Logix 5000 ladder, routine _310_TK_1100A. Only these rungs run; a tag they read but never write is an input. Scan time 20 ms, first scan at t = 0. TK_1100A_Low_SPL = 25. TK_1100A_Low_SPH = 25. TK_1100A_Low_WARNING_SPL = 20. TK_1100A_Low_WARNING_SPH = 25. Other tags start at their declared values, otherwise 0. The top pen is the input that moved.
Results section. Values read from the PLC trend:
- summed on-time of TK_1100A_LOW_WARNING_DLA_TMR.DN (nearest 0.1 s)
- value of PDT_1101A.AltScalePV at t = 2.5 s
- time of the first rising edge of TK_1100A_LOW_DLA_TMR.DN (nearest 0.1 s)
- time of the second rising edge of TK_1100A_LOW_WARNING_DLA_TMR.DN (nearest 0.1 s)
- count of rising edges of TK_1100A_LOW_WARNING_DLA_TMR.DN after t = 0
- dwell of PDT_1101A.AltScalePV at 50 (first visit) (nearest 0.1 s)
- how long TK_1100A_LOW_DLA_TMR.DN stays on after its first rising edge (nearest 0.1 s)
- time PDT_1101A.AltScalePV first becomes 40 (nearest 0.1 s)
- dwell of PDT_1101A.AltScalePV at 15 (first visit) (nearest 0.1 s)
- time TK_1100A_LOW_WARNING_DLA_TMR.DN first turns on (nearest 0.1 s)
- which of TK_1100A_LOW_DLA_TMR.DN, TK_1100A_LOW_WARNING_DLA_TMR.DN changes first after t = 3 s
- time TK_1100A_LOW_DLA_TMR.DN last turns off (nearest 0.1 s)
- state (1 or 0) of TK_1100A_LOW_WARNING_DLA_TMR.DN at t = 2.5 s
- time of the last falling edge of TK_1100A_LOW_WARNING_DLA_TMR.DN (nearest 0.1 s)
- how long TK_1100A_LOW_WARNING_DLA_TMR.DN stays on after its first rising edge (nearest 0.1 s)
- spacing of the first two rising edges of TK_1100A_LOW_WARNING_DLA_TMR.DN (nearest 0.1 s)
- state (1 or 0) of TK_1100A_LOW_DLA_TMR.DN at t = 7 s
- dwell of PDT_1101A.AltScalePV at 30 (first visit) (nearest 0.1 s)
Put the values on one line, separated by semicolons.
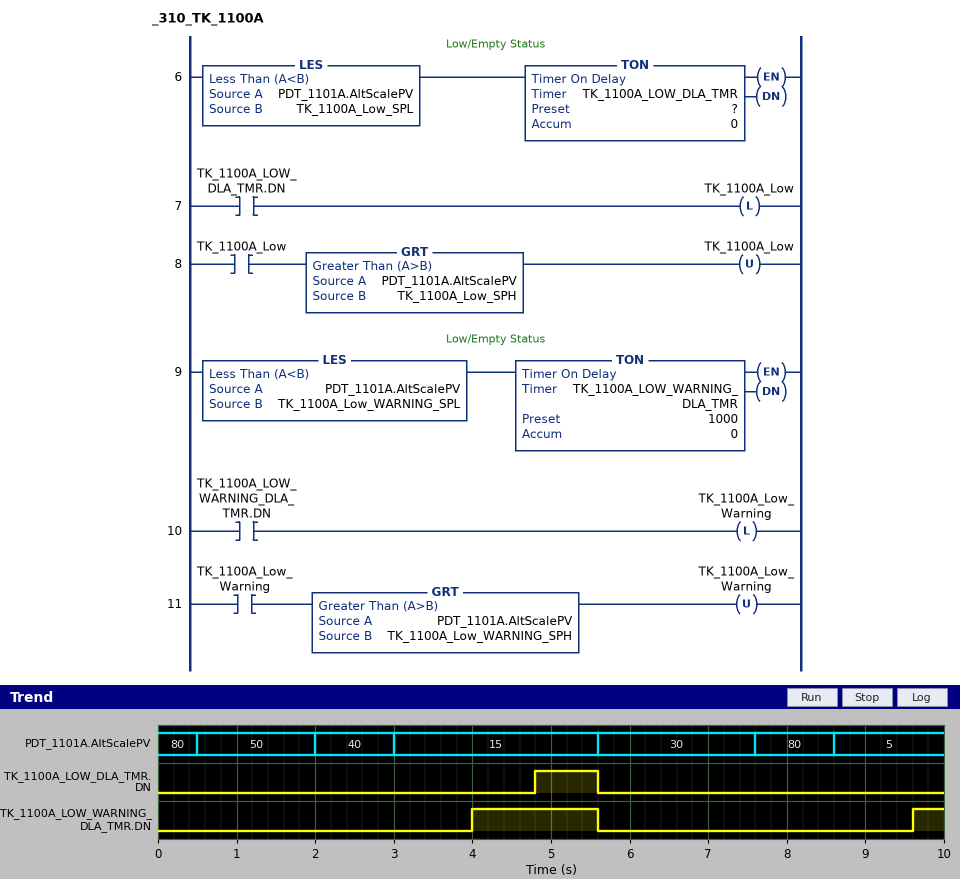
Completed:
2.0 s; 40; 4.8 s; 9.6 s; 2; 1.5 s; 0.8 s; 2.0 s; 2.6 s; 4.0 s; TK_1100A_LOW_WARNING_DLA_TMR.DN; 5.6 s; 0; 5.6 s; 1.6 s; 5.6 s; 0; 2.0 s
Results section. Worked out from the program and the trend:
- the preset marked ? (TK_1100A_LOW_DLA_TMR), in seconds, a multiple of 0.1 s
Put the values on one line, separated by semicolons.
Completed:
1.8 s
